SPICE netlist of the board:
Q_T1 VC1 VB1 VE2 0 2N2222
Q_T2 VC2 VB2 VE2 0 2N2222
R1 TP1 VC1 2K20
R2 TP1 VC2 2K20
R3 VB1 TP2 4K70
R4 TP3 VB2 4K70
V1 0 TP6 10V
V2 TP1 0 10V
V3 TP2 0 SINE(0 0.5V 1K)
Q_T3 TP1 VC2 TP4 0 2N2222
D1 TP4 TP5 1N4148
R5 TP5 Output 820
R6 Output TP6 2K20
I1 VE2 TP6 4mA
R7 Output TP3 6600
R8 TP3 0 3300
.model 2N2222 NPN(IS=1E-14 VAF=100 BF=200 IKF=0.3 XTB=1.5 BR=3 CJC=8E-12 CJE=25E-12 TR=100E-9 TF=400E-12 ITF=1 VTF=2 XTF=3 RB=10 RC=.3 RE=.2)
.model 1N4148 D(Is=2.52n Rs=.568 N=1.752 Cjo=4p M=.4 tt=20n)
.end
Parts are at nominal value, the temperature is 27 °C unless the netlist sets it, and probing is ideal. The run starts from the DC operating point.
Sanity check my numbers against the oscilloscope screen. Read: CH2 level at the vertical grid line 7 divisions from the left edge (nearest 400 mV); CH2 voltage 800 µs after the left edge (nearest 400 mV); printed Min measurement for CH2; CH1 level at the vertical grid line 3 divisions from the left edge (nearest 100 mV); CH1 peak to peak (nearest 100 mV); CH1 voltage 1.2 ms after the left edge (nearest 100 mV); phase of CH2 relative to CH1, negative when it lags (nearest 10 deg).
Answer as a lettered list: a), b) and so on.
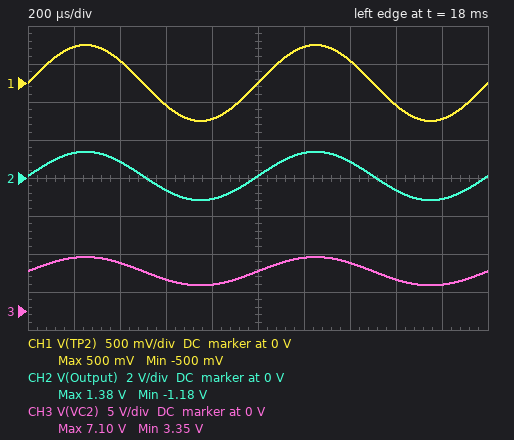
a) 800 mV
b) -1.2 V
c) -1.18 V
d) -300 mV
e) 1.0 V
f) 500 mV
g) 0 deg
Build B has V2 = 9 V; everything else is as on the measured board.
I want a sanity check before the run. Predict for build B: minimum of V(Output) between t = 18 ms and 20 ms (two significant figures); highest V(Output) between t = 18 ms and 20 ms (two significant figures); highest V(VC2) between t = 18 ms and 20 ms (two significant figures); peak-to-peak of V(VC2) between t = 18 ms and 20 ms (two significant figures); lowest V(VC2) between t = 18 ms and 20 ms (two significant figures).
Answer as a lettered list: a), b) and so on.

a) -1.3 V
b) 1.3 V
c) 6.9 V
d) 3.7 V
e) 3.2 V
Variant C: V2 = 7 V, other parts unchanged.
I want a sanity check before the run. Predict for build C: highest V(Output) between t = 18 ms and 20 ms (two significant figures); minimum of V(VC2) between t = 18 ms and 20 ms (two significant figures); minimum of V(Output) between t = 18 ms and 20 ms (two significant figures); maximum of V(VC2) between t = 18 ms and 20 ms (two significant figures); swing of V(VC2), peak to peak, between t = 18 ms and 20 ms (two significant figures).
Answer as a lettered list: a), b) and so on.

a) 440 mV
b) 2.9 V
c) -1.5 V
d) 5.7 V
e) 2.8 V
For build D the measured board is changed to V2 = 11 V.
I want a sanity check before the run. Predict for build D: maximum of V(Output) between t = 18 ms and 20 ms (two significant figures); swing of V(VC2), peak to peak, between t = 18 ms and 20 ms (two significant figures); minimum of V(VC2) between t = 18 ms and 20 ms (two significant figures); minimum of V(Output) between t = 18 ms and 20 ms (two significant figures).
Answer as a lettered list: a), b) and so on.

a) 1.5 V
b) 3.7 V
c) 3.5 V
d) -1.1 V
